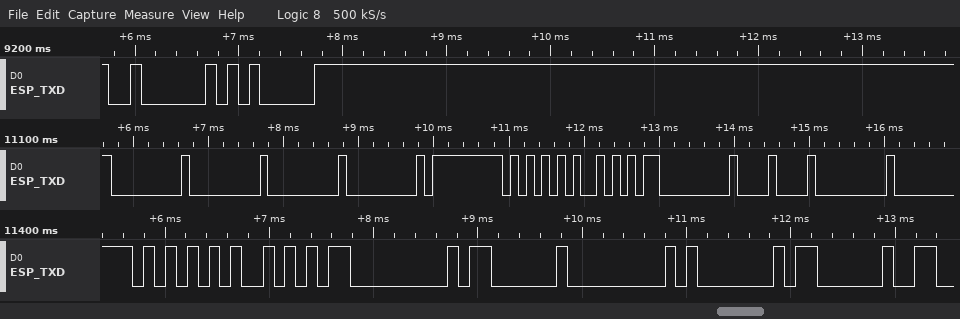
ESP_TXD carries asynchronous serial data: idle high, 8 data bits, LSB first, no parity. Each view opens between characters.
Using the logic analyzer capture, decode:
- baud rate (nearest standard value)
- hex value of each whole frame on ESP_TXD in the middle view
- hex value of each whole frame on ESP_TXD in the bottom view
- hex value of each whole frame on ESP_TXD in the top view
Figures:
9600 baud
00, 00, 00, 00, FF, 55, AA, 00, 08, 00
55, AA, 00, 03, 00, 01, 03
02, 05
